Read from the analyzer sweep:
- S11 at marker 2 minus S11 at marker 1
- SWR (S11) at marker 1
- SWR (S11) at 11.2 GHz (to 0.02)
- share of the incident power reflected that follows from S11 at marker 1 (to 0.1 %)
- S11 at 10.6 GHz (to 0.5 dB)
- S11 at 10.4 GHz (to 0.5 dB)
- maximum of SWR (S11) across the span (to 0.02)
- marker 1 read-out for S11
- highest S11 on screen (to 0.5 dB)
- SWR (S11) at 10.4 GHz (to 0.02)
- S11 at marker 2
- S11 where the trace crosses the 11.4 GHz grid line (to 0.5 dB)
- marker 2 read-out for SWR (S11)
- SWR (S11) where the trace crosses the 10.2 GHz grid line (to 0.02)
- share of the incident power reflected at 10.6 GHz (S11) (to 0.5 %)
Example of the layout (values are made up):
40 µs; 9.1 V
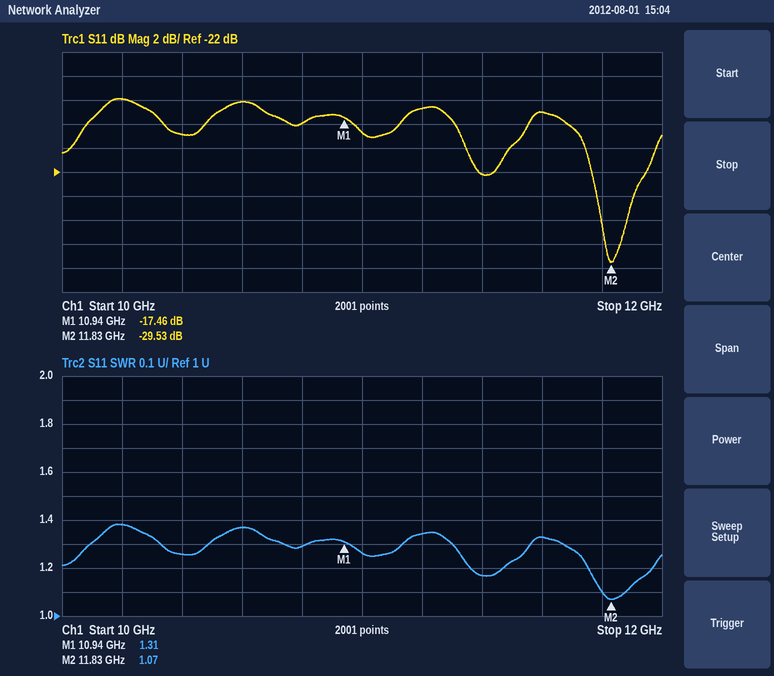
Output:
-12.07 dB; 1.31; 1.34; 1.8 %; -16.0 dB; -19.0 dB; 1.38; -17.46 dB; -16.0 dB; 1.26; -29.53 dB; -22.0 dB; 1.07; 1.38; 2.5 %
